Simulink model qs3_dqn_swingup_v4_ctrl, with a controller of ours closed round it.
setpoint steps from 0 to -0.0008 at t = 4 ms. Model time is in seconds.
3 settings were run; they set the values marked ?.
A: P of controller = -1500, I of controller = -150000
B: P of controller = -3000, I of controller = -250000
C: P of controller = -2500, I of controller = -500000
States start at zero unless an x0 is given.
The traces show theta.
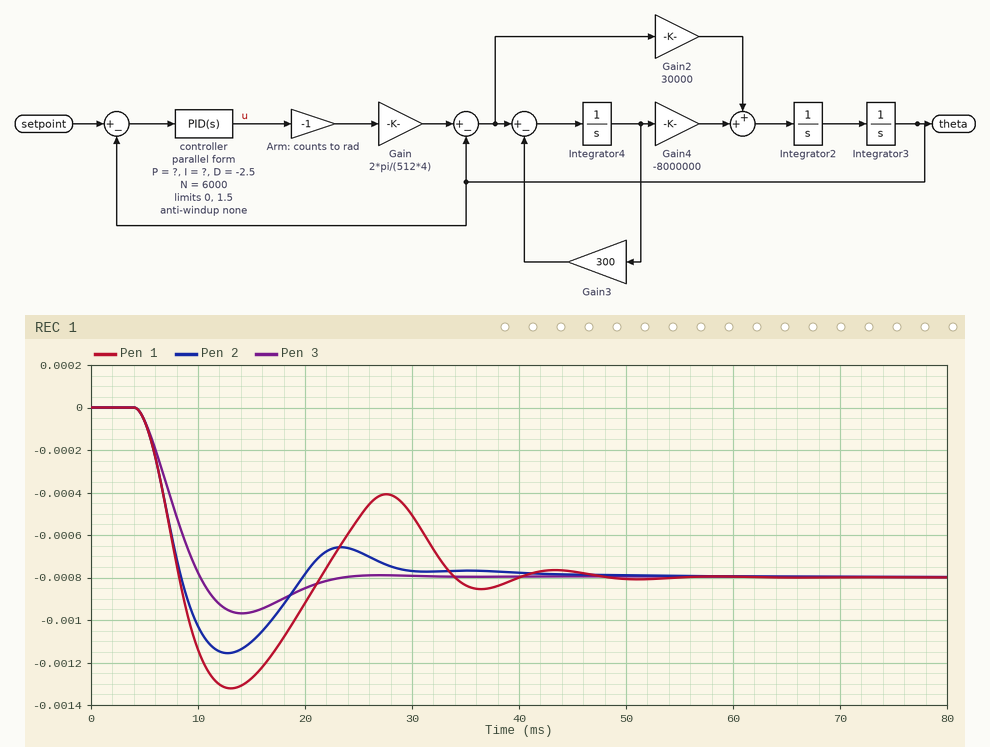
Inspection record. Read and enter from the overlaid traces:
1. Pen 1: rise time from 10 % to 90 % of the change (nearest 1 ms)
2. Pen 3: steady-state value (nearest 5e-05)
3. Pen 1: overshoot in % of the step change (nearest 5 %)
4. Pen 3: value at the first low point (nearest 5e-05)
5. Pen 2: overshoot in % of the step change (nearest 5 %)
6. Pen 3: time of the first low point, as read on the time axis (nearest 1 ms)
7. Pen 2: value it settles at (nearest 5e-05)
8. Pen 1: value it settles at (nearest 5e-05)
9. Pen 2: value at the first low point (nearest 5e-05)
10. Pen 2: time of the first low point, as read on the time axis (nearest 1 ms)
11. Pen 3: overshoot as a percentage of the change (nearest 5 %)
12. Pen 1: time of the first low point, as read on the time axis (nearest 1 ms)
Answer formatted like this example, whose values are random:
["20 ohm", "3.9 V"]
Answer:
["3 ms", "-0.00080", "65 %", "-0.00095", "45 %", "14 ms", "-0.00080", "-0.00080", "-0.00115", "13 ms", "20 %", "13 ms"]
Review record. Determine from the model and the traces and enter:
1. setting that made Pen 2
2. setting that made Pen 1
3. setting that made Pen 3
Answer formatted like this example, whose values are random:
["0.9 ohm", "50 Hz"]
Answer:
["B", "C", "A"]
